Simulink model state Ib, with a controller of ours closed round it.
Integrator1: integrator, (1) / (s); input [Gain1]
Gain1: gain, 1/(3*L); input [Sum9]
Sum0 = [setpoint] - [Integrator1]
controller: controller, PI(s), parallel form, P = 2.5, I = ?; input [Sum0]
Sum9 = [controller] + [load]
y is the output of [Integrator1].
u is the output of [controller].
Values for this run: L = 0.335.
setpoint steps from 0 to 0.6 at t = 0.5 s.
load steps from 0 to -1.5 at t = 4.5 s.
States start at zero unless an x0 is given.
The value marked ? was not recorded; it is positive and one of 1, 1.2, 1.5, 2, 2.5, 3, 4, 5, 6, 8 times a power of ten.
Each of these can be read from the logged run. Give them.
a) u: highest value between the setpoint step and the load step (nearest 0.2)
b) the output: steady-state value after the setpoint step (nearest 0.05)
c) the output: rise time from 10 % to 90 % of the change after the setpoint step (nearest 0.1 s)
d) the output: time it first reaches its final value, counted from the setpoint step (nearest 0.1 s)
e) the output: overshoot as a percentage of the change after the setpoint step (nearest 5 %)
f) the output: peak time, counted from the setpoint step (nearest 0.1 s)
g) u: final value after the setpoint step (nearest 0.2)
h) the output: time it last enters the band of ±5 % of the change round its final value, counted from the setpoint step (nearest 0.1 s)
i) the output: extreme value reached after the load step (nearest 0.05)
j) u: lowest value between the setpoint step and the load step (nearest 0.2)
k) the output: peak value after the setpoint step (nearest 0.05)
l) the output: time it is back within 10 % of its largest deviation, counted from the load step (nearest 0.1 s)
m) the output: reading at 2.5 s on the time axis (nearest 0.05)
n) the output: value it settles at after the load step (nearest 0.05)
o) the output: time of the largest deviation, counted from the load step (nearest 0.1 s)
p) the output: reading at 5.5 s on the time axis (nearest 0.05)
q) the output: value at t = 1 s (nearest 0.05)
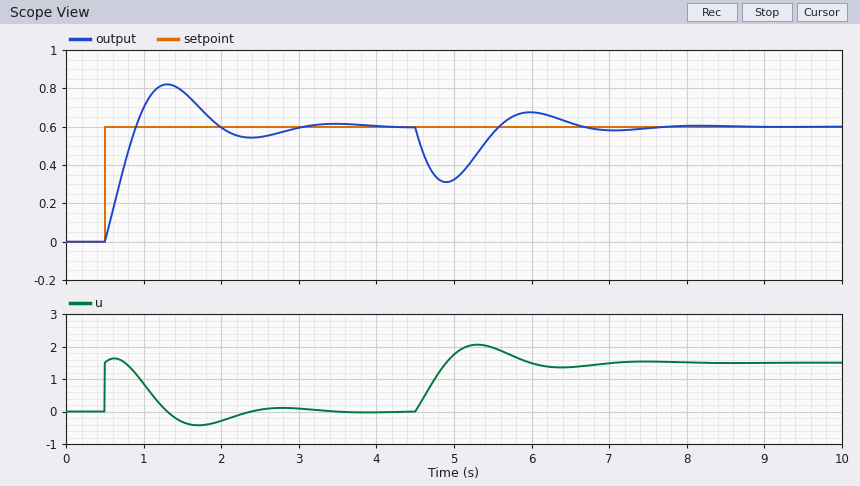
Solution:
1.6
0.60
0.3 s
0.4 s
35 %
0.8 s
0.0
2.3 s
0.30
-0.4
0.80
1.9 s
0.55
0.60
0.4 s
0.55
0.70
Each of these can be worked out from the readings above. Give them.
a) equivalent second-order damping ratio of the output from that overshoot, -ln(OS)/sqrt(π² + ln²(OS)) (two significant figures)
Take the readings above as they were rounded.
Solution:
0.32
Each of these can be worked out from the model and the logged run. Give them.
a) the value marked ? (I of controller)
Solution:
10
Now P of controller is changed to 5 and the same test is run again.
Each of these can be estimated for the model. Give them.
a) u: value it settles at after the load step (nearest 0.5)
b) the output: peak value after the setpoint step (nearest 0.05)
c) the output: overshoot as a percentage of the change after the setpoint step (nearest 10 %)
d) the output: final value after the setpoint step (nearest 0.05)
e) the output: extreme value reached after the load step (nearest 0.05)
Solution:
1.5
0.70
20 %
0.60
0.40
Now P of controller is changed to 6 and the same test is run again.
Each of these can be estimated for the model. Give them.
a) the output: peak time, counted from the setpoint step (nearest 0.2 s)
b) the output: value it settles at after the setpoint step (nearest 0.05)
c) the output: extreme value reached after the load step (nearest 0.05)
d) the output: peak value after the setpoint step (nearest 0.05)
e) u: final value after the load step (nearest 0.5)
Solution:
0.6 s
0.60
0.40
0.70
1.5
